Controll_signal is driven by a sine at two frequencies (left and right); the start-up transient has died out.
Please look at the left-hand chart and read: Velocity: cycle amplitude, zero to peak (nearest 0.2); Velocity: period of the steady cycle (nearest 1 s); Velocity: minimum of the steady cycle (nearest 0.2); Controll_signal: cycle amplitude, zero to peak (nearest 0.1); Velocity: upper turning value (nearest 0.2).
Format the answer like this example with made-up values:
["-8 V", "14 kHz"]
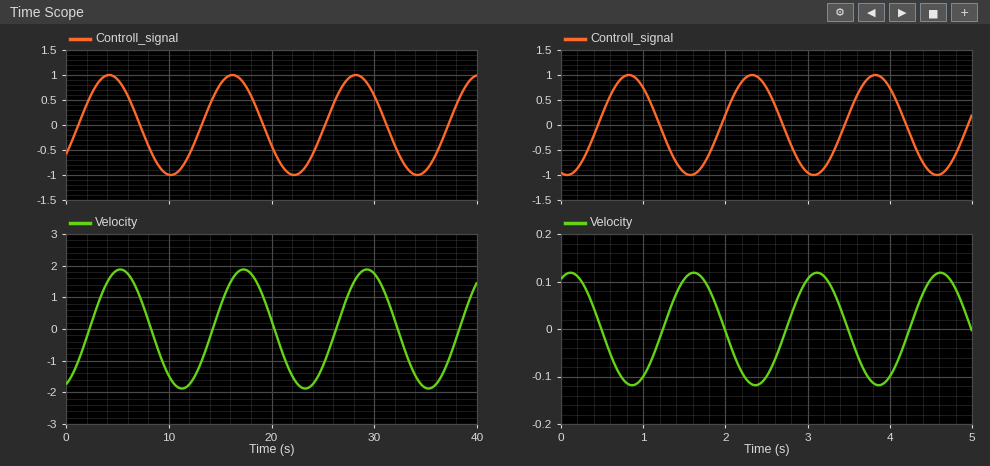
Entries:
["1.8", "12 s", "-1.8", "1.0", "1.8"]
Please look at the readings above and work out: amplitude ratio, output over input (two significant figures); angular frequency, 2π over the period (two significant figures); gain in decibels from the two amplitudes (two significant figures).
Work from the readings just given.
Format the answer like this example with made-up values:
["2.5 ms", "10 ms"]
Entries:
["1.8", "0.52 rad/s", "5.1 dB"]
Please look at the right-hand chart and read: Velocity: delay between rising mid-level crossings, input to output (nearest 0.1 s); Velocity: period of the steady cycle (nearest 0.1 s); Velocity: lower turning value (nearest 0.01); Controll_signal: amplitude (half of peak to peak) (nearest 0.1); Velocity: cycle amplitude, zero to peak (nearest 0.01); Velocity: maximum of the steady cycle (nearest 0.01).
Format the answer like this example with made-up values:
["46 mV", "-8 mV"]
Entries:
["0.8 s", "1.5 s", "-0.12", "1.0", "0.12", "0.12"]
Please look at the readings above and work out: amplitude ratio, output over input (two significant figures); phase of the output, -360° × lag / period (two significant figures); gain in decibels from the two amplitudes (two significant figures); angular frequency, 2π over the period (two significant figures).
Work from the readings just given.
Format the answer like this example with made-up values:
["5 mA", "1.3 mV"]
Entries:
["0.12", "-190°", "-18 dB", "4.2 rad/s"]
